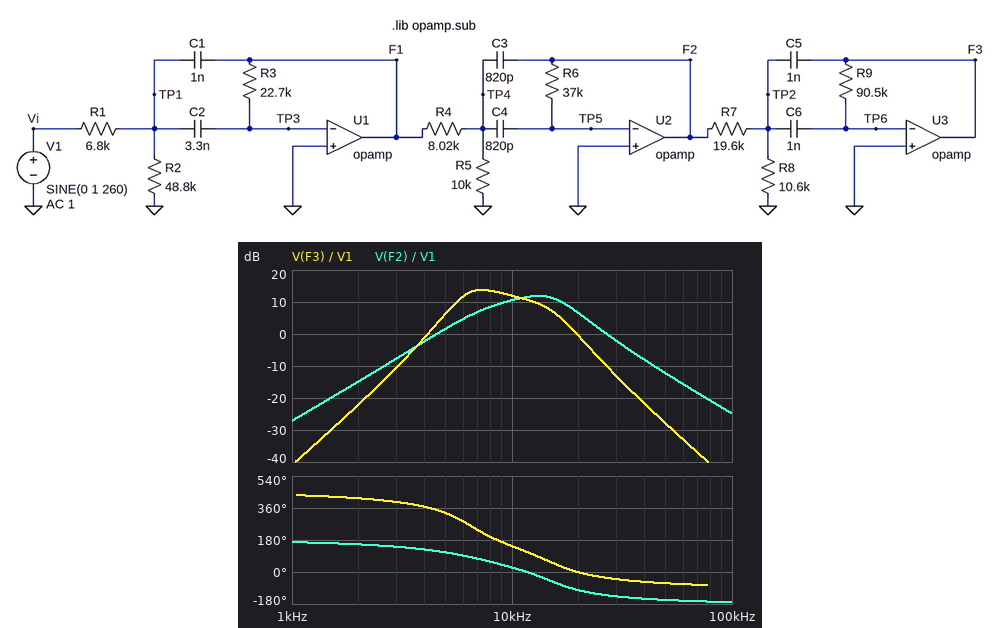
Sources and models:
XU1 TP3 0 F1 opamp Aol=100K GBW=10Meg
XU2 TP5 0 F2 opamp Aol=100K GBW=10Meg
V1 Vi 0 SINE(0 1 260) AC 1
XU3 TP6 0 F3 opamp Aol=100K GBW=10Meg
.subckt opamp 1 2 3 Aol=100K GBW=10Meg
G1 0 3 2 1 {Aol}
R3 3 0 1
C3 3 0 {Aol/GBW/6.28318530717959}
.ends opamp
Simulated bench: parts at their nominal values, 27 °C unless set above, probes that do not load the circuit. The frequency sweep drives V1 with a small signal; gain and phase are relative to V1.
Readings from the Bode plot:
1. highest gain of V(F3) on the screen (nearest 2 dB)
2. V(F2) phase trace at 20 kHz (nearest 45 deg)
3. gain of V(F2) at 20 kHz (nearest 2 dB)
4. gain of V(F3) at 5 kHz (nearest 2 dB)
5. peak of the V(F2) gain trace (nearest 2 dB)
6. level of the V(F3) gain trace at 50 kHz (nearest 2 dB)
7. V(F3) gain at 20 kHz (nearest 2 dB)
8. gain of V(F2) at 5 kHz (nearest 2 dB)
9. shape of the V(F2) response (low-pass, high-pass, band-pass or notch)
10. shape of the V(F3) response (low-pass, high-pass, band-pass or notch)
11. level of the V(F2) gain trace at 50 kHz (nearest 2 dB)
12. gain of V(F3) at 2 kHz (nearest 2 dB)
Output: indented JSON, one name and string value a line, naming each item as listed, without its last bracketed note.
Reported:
{
  "highest gain of V(F3) on the screen": "14 dB",
  "V(F2) phase trace at 20 kHz": "-90 deg",
  "gain of V(F2) at 20 kHz": "6 dB",
  "gain of V(F3) at 5 kHz": "6 dB",
  "peak of the V(F2) gain trace": "12 dB",
  "level of the V(F3) gain trace at 50 kHz": "-28 dB",
  "V(F3) gain at 20 kHz": "0 dB",
  "gain of V(F2) at 5 kHz": "2 dB",
  "shape of the V(F2) response": "band-pass",
  "shape of the V(F3) response": "band-pass",
  "level of the V(F2) gain trace at 50 kHz": "-12 dB",
  "gain of V(F3) at 2 kHz": "-22 dB"
}
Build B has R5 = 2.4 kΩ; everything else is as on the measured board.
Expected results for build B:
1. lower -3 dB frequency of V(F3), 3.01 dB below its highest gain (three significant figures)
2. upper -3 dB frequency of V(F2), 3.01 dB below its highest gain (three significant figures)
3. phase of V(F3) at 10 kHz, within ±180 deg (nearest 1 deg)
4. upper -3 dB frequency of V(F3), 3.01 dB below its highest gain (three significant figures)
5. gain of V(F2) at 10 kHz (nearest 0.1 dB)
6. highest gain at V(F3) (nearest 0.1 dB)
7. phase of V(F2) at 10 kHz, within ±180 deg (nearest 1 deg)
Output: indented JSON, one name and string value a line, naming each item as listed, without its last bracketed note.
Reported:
{
  "lower -3 dB frequency of V(F3), 3.01 dB below its highest gain": "5.70 kHz",
  "upper -3 dB frequency of V(F2), 3.01 dB below its highest gain": "26.9 kHz",
  "phase of V(F3) at 10 kHz, within ±180 deg": "172 deg",
  "upper -3 dB frequency of V(F3), 3.01 dB below its highest gain": "10.8 kHz",
  "gain of V(F2) at 10 kHz": "1.7 dB",
  "highest gain at V(F3)": "5.4 dB",
  "phase of V(F2) at 10 kHz, within ±180 deg": "51 deg"
}
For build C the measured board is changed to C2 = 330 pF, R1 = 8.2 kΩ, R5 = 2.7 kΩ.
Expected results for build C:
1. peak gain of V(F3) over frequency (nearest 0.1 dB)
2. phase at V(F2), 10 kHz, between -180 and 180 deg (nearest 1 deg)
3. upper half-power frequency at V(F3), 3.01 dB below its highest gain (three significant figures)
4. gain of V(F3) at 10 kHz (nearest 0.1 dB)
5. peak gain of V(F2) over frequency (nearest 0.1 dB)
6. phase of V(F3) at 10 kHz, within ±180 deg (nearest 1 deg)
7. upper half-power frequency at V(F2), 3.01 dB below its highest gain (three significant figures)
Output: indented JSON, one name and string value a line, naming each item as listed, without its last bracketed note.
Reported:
{
  "peak gain of V(F3) over frequency": "-3.9 dB",
  "phase at V(F2), 10 kHz, between -180 and 180 deg": "129 deg",
  "upper half-power frequency at V(F3), 3.01 dB below its highest gain": "25.5 kHz",
  "gain of V(F3) at 10 kHz": "-11.1 dB",
  "peak gain of V(F2) over frequency": "4.0 dB",
  "phase of V(F3) at 10 kHz, within ±180 deg": "-111 deg",
  "upper half-power frequency at V(F2), 3.01 dB below its highest gain": "27.4 kHz"
}
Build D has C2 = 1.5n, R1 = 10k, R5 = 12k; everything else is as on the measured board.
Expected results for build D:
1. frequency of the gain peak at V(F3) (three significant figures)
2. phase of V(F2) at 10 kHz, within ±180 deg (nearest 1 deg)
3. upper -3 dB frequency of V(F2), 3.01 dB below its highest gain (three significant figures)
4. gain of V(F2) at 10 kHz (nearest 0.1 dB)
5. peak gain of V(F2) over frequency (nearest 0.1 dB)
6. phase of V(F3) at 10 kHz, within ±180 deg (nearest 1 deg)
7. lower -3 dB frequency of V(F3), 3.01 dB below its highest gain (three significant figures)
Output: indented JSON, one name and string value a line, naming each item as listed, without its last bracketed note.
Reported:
{
  "frequency of the gain peak at V(F3)": "8.00 kHz",
  "phase of V(F2) at 10 kHz, within ±180 deg": "41 deg",
  "upper -3 dB frequency of V(F2), 3.01 dB below its highest gain": "17.6 kHz",
  "gain of V(F2) at 10 kHz": "6.6 dB",
  "peak gain of V(F2) over frequency": "8.5 dB",
  "phase of V(F3) at 10 kHz, within ±180 deg": "162 deg",
  "lower -3 dB frequency of V(F3), 3.01 dB below its highest gain": "5.98 kHz"
}
